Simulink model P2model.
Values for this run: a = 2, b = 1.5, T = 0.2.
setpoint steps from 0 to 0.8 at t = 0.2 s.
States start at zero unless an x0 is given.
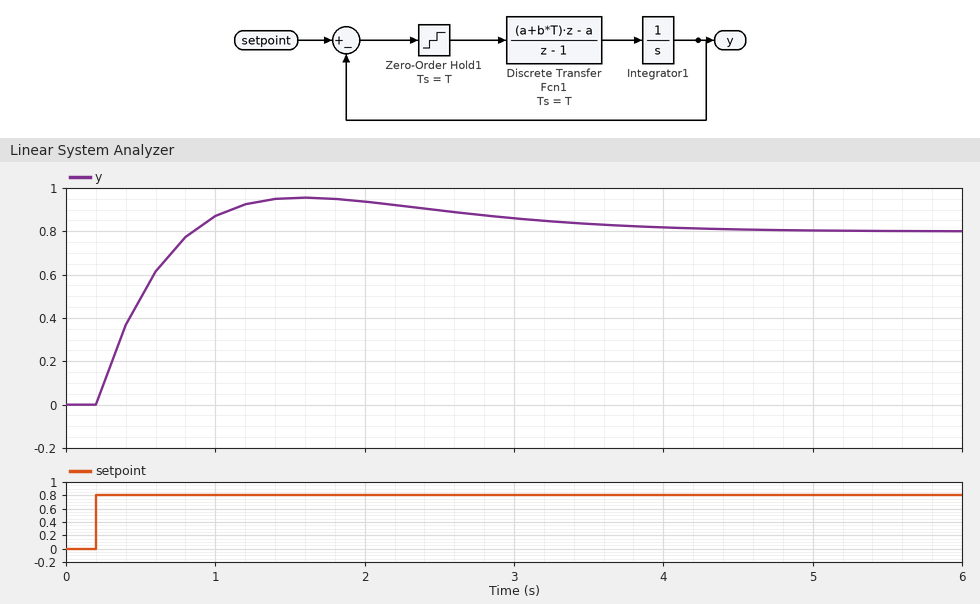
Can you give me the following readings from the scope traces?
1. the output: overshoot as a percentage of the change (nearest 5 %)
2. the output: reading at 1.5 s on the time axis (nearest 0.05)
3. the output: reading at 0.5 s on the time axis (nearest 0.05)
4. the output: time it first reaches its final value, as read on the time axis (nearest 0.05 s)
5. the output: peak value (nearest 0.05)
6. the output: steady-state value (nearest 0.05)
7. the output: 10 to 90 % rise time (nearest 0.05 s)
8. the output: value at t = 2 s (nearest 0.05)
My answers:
20 %
0.95
0.50
0.85 s
0.95
0.80
0.50 s
0.95
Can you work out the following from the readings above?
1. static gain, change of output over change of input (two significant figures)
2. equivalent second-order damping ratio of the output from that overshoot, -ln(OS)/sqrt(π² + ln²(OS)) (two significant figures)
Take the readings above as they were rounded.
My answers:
1.0
0.46
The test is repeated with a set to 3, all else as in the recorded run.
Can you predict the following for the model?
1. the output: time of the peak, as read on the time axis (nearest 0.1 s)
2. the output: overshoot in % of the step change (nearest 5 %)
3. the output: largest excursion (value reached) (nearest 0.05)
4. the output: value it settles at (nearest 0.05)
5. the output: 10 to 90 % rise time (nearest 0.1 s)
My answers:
1.2 s
10 %
0.90
0.80
0.3 s
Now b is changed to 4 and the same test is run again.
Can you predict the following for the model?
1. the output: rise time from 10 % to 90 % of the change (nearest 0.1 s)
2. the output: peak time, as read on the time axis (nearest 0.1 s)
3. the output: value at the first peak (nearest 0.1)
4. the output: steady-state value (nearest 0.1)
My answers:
0.3 s
1.2 s
1.1
0.8
